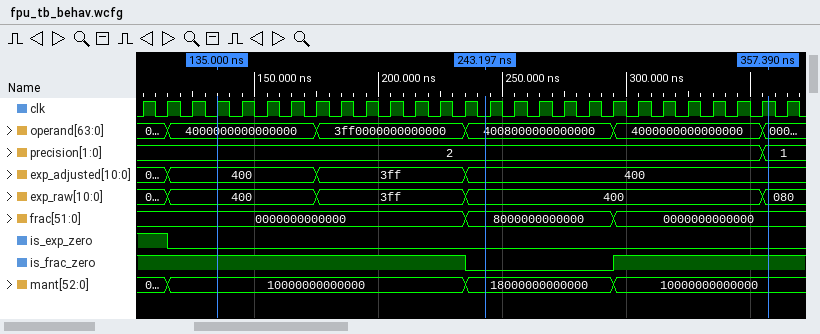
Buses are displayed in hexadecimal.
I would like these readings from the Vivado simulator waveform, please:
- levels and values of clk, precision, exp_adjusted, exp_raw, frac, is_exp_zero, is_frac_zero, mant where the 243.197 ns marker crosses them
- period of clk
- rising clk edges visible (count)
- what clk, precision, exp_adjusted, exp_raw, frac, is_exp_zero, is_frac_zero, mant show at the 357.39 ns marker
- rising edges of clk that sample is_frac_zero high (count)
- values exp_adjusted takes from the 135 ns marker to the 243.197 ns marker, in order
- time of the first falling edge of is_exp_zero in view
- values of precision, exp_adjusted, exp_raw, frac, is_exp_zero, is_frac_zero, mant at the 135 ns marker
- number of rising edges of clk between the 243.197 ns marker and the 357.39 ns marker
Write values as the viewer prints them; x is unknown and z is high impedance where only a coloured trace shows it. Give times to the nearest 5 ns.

clk=0, precision=2, exp_adjusted=400, exp_raw=400, frac=8000000000000, is_exp_zero=0, is_frac_zero=0, mant=18000000000000
10 ns
27
clk=1, precision=1, exp_adjusted=400, exp_raw=080, frac=0000000000000, is_exp_zero=0, is_frac_zero=1, mant=10000000000000
21
400, 3ff, 400
115 ns
precision=2, exp_adjusted=400, exp_raw=400, frac=0000000000000, is_exp_zero=0, is_frac_zero=1, mant=10000000000000
12
